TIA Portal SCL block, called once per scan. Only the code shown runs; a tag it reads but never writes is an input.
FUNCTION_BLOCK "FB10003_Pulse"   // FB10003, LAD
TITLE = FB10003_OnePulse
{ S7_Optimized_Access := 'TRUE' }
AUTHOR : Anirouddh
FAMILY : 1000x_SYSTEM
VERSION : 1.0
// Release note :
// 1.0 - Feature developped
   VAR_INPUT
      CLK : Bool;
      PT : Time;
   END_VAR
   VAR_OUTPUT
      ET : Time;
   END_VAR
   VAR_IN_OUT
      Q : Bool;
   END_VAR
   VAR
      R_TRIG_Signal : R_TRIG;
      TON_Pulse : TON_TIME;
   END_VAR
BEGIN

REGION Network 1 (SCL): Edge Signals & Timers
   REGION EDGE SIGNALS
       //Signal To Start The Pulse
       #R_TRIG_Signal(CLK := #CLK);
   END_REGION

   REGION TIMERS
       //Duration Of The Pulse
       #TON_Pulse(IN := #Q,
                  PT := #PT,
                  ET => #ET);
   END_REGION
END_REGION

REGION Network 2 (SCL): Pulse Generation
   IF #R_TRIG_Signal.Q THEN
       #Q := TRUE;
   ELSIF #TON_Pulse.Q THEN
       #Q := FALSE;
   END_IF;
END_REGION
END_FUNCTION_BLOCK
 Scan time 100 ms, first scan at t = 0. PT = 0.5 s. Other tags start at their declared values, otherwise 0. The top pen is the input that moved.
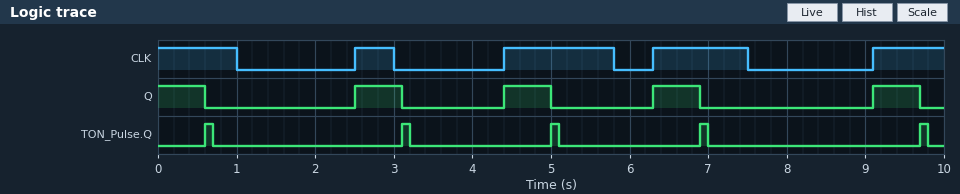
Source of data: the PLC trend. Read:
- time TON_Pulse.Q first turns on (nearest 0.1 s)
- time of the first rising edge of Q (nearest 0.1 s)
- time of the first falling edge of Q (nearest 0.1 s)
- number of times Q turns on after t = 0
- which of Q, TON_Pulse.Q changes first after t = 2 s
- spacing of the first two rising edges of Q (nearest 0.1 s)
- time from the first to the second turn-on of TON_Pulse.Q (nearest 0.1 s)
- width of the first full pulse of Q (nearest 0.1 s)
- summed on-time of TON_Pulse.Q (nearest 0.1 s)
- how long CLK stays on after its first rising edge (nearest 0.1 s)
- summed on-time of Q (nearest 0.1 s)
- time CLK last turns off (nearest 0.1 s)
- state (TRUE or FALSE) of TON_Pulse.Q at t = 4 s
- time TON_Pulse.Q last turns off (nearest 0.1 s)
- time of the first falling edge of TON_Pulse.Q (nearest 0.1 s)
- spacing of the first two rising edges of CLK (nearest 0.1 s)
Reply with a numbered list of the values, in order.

1. 0.6 s
2. 2.5 s
3. 0.6 s
4. 4
5. Q
6. 1.9 s
7. 2.5 s
8. 0.6 s
9. 0.5 s
10. 0.5 s
11. 3.0 s
12. 7.5 s
13. FALSE
14. 9.8 s
15. 0.7 s
16. 1.9 s
